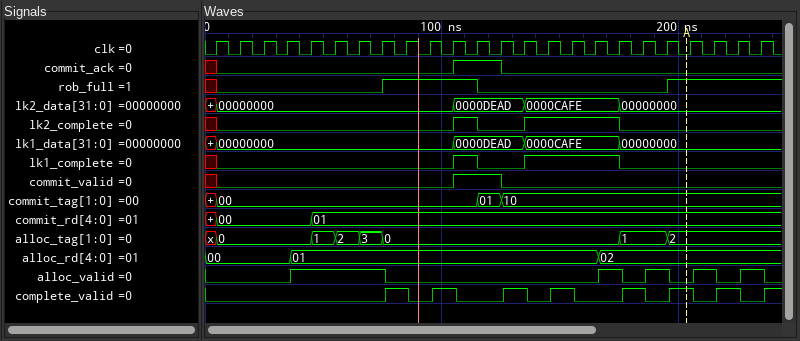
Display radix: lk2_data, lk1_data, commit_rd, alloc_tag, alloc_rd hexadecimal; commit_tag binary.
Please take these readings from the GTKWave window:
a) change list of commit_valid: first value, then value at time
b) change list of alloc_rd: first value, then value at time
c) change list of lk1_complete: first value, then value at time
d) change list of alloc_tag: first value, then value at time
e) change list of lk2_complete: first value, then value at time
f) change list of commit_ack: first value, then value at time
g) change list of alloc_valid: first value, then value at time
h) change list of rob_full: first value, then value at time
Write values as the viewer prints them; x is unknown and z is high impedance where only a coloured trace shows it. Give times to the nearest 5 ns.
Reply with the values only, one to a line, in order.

x, 0 at 5 ns, 1 at 105 ns, 0 at 125 ns
00, 01 at 35 ns, 02 at 165 ns
x, 0 at 5 ns, 1 at 105 ns, 0 at 115 ns, 1 at 135 ns, 0 at 175 ns
x, 0 at 5 ns, 1 at 45 ns, 2 at 55 ns, 3 at 65 ns, 0 at 75 ns, 1 at 175 ns, 2 at 195 ns
x, 0 at 5 ns, 1 at 105 ns, 0 at 115 ns, 1 at 135 ns, 0 at 175 ns
x, 0 at 5 ns, 1 at 105 ns, 0 at 125 ns
0, 1 at 35 ns, 0 at 75 ns, 1 at 165 ns, 0 at 175 ns, 1 at 185 ns, 0 at 195 ns, 1 at 205 ns, 0 at 215 ns, 1 at 225 ns, 0 at 235 ns
x, 0 at 5 ns, 1 at 75 ns, 0 at 115 ns, 1 at 195 ns
